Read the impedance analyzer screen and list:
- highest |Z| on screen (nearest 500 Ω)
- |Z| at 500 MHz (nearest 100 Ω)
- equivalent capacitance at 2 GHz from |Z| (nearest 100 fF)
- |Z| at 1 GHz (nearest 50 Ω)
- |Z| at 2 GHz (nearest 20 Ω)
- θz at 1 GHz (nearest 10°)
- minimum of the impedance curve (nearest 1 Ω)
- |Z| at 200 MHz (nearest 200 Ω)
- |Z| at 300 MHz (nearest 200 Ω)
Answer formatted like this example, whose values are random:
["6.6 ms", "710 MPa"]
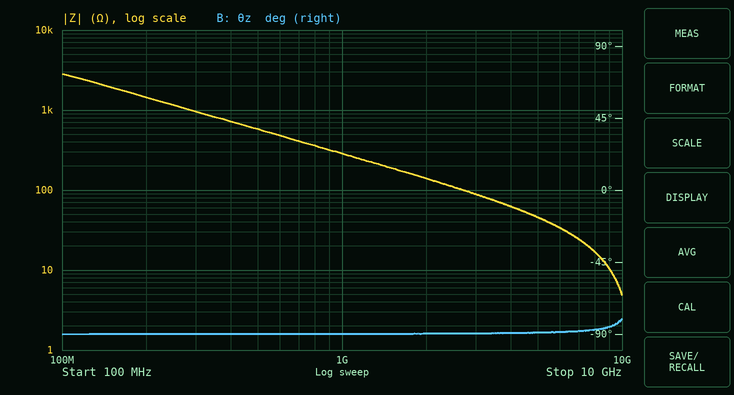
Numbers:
["3.0 kΩ", "600 Ω", "600 fF", "300 Ω", "140 Ω", "-90°", "5 Ω", "1.4 kΩ", "1.0 kΩ"]
